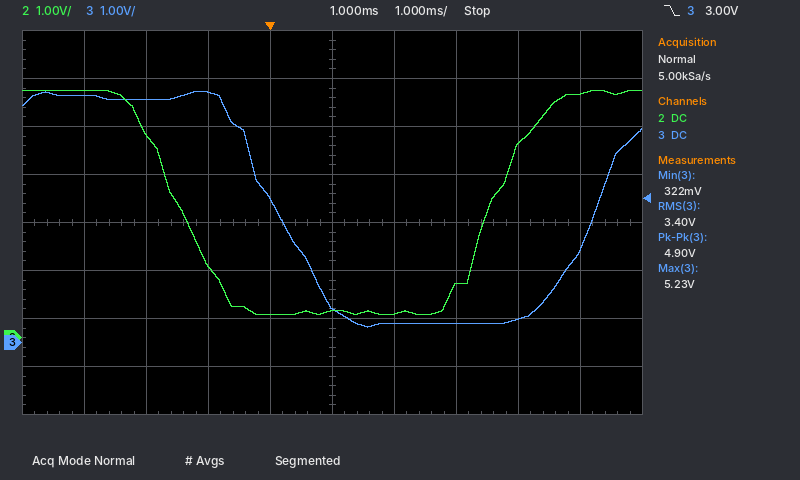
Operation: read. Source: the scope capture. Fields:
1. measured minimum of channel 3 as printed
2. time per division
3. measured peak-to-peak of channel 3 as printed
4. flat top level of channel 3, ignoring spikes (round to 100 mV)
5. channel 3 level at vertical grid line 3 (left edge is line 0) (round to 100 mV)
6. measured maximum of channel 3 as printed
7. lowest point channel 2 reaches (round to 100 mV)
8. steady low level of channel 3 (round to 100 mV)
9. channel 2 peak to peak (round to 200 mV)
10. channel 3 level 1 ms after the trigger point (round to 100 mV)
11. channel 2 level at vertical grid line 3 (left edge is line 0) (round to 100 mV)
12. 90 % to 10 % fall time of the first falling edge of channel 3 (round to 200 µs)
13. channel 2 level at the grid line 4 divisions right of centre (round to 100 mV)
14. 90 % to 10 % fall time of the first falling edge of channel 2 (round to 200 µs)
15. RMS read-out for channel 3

322 mV
1 ms
4.90 V
5.1 V
5.2 V
5.23 V
500 mV
400 mV
4.6 V
700 mV
1.5 V
1.6 ms
5.1 V
1.4 ms
3.40 V
